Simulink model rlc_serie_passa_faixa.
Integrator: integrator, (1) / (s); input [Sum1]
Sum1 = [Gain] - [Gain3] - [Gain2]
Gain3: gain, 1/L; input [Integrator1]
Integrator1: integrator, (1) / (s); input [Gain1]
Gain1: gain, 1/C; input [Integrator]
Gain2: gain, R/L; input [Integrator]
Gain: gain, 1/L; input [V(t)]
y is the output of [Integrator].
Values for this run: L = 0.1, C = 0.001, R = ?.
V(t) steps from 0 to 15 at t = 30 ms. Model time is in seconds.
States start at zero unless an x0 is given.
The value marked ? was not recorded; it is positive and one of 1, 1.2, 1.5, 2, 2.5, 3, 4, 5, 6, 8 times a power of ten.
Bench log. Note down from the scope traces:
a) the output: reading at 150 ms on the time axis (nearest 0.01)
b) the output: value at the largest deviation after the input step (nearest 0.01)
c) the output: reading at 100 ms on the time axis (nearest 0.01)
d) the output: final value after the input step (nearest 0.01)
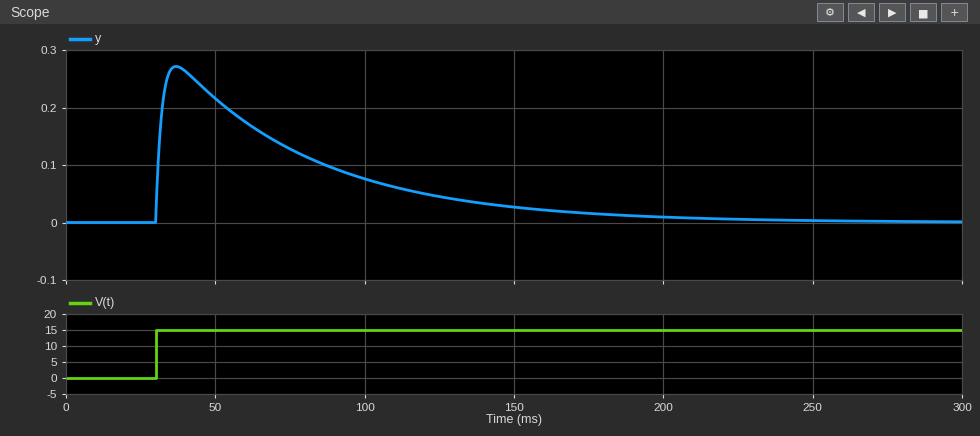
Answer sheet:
0.03
0.27
0.08
0.00
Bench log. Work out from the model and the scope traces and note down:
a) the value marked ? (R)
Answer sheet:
50
